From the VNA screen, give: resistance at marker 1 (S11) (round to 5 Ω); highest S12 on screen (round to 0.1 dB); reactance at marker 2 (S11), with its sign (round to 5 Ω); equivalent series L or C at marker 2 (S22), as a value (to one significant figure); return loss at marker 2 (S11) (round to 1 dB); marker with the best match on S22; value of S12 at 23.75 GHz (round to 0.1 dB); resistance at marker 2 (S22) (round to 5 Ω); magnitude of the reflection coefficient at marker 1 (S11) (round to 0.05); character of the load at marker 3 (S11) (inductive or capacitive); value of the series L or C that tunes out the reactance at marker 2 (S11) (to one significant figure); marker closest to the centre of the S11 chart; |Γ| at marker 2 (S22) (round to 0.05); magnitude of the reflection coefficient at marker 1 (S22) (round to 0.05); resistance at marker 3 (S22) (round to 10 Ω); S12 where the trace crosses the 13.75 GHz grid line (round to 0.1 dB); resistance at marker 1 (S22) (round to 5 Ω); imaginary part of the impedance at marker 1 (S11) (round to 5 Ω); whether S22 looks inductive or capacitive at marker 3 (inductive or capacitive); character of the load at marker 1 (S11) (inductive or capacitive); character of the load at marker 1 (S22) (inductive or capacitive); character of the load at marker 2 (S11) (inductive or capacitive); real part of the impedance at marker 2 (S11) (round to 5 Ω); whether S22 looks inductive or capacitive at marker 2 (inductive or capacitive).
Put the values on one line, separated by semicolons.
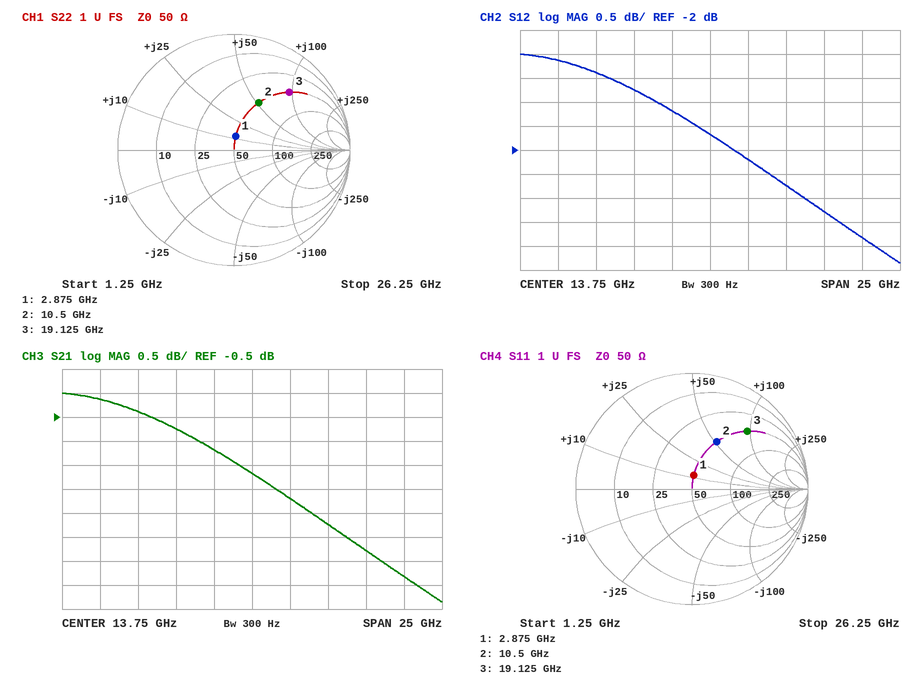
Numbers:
50 Ω; 0.0 dB; +50 Ω; 800 pH; 7 dB; marker 1; -3.8 dB; 50 Ω; 0.10; inductive; 300 fF; marker 1; 0.45; 0.10; 50 Ω; -1.7 dB; 50 Ω; +10 Ω; inductive; inductive; inductive; inductive; 50 Ω; inductive
